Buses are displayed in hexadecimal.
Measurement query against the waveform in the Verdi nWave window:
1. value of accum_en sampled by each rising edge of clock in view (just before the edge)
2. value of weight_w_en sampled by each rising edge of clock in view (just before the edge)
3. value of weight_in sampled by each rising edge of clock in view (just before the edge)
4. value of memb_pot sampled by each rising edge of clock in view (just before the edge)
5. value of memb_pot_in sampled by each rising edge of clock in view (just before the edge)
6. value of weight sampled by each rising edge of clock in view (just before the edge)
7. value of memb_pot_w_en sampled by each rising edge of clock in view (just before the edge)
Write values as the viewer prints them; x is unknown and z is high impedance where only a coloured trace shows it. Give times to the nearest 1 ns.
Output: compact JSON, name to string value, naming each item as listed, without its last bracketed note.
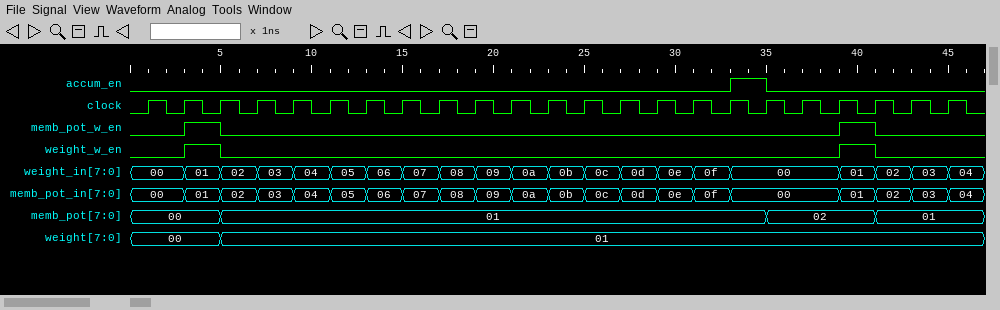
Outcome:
{"value of accum_en sampled by each rising edge of clock in view": "0 0 0 0 0 0 0 0 0 0 0 0 0 0 0 0 0 1 0 0 0 0 0", "value of weight_w_en sampled by each rising edge of clock in view": "0 0 1 0 0 0 0 0 0 0 0 0 0 0 0 0 0 0 0 0 1 0 0", "value of weight_in sampled by each rising edge of clock in view": "00, 00, 01, 02, 03, 04, 05, 06, 07, 08, 09, 0a, 0b, 0c, 0d, 0e, 0f, 00, 00, 00, 01, 02, 03", "value of memb_pot sampled by each rising edge of clock in view": "00, 00, 00, 01, 01, 01, 01, 01, 01, 01, 01, 01, 01, 01, 01, 01, 01, 01, 02, 02, 02, 01, 01", "value of memb_pot_in sampled by each rising edge of clock in view": "00, 00, 01, 02, 03, 04, 05, 06, 07, 08, 09, 0a, 0b, 0c, 0d, 0e, 0f, 00, 00, 00, 01, 02, 03", "value of weight sampled by each rising edge of clock in view": "00, 00, 00, 01, 01, 01, 01, 01, 01, 01, 01, 01, 01, 01, 01, 01, 01, 01, 01, 01, 01, 01, 01", "value of memb_pot_w_en sampled by each rising edge of clock in view": "0 0 1 0 0 0 0 0 0 0 0 0 0 0 0 0 0 0 0 0 1 0 0"}
